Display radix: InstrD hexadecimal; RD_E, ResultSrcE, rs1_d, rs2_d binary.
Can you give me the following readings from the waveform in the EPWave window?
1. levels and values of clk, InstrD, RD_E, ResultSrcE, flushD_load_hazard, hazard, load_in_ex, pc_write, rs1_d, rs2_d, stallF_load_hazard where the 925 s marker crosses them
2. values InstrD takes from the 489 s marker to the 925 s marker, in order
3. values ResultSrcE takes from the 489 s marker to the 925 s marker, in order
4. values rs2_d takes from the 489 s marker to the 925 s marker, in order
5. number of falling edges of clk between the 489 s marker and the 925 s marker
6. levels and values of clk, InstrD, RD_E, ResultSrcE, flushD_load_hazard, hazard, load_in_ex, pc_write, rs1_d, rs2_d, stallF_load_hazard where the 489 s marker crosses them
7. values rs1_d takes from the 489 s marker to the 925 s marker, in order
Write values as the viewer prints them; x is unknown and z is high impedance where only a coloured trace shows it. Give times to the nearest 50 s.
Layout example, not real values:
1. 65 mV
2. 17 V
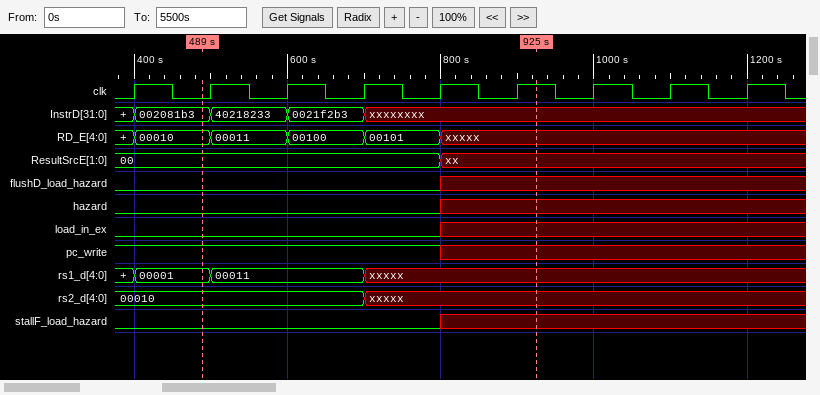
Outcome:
1. clk=1, InstrD=xxxxxxxx, RD_E=xxxxx, ResultSrcE=xx, flushD_load_hazard=x, hazard=x, load_in_ex=x, pc_write=x, rs1_d=xxxxx, rs2_d=xxxxx, stallF_load_hazard=x
2. 002081b3, 40218233, 0021f2b3, xxxxxxxx
3. 00, xx
4. 00010, xxxxx
5. 4
6. clk=0, InstrD=002081b3, RD_E=00010, ResultSrcE=00, flushD_load_hazard=0, hazard=0, load_in_ex=0, pc_write=1, rs1_d=00001, rs2_d=00010, stallF_load_hazard=0
7. 00001, 00011, xxxxx
